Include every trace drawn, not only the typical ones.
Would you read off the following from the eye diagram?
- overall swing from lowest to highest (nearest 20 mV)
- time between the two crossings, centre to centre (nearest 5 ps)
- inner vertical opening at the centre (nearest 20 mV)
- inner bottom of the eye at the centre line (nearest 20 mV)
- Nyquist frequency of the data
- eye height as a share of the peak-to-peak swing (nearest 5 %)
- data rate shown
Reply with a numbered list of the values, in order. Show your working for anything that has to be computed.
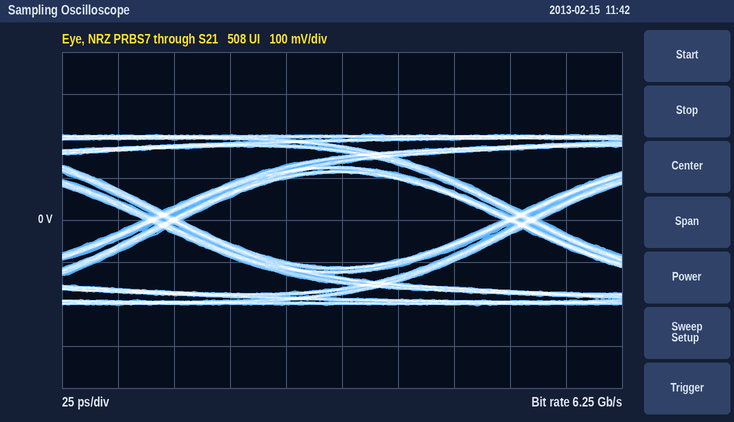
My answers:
1. 400 mV
2. 160 ps
3. 220 mV
4. -120 mV
5. 3.125 GHz
6. 220 mV / 400 mV ≈ 55 %
7. 6.25 Gb/s
